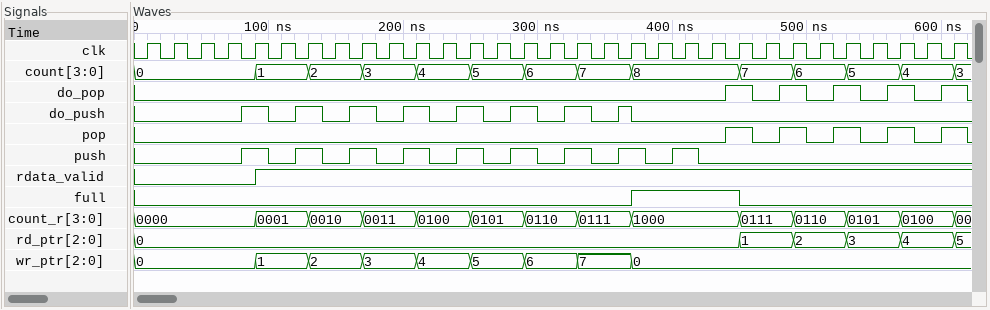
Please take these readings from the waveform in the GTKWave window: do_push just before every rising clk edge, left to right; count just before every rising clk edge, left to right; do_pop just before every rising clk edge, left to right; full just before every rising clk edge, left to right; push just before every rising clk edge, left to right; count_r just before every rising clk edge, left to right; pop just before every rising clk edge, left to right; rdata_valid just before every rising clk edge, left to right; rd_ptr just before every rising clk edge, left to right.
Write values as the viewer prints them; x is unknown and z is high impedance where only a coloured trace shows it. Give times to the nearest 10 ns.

0 0 0 0 1 0 1 0 1 0 1 0 1 0 1 0 1 0 1 0 0 0 0 0 0 0 0 0 0 0 0
0, 0, 0, 0, 0, 1, 1, 2, 2, 3, 3, 4, 4, 5, 5, 6, 6, 7, 7, 8, 8, 8, 8, 7, 7, 6, 6, 5, 5, 4, 4
0 0 0 0 0 0 0 0 0 0 0 0 0 0 0 0 0 0 0 0 0 0 1 0 1 0 1 0 1 0 1
0 0 0 0 0 0 0 0 0 0 0 0 0 0 0 0 0 0 0 1 1 1 1 0 0 0 0 0 0 0 0
0 0 0 0 1 0 1 0 1 0 1 0 1 0 1 0 1 0 1 0 1 0 0 0 0 0 0 0 0 0 0
0000, 0000, 0000, 0000, 0000, 0001, 0001, 0010, 0010, 0011, 0011, 0100, 0100, 0101, 0101, 0110, 0110, 0111, 0111, 1000, 1000, 1000, 1000, 0111, 0111, 0110, 0110, 0101, 0101, 0100, 0100
0 0 0 0 0 0 0 0 0 0 0 0 0 0 0 0 0 0 0 0 0 0 1 0 1 0 1 0 1 0 1
0 0 0 0 0 1 1 1 1 1 1 1 1 1 1 1 1 1 1 1 1 1 1 1 1 1 1 1 1 1 1
0, 0, 0, 0, 0, 0, 0, 0, 0, 0, 0, 0, 0, 0, 0, 0, 0, 0, 0, 0, 0, 0, 0, 1, 1, 2, 2, 3, 3, 4, 4
